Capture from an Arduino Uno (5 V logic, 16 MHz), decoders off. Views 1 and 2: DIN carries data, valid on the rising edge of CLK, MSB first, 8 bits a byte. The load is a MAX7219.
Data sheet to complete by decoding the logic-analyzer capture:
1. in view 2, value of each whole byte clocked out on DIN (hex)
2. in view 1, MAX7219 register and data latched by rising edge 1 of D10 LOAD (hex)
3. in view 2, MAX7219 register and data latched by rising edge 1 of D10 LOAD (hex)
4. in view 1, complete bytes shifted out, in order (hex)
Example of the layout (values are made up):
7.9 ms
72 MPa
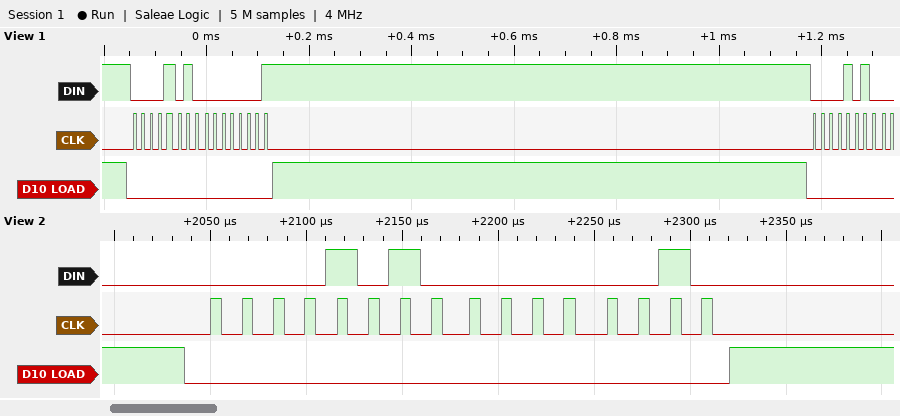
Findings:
0A 02
register 0xA, data 0x01
register 0xA, data 0x02
0A 01 0A
